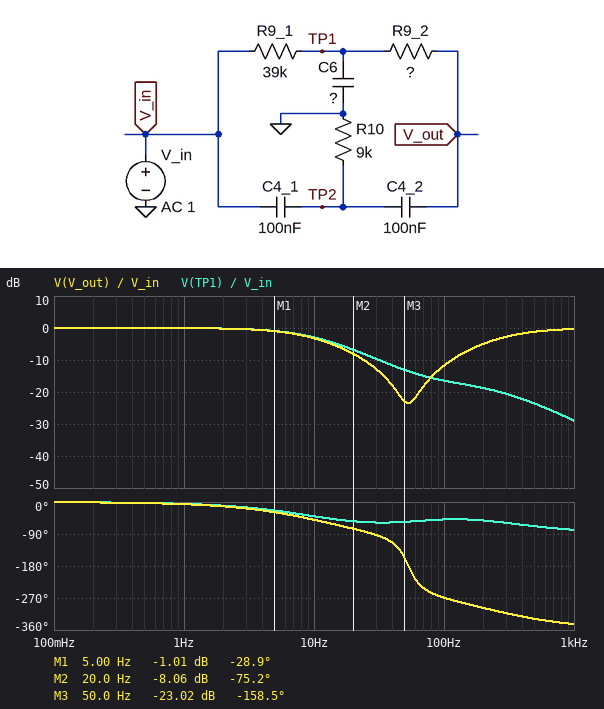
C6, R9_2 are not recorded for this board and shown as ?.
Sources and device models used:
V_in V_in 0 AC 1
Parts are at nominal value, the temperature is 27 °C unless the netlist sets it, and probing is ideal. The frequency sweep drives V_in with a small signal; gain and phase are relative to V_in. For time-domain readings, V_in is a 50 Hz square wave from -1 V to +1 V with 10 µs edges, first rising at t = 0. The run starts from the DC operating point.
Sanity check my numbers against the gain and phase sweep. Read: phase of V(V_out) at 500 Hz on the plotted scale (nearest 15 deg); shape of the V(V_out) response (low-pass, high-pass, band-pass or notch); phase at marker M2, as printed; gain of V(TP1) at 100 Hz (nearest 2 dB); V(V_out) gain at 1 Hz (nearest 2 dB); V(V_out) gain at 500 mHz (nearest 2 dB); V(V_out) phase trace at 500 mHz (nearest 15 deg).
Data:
-330 deg
notch
-75.2 deg
-16 dB
0 dB
0 dB
0 deg
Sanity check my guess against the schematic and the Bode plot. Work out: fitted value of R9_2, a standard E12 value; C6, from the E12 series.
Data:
27 kΩ
270 nF
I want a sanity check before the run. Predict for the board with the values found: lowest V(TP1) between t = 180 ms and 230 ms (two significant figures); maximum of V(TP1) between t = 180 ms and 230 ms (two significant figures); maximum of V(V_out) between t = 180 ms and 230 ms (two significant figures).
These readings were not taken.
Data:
-360 mV
360 mV
1.8 V
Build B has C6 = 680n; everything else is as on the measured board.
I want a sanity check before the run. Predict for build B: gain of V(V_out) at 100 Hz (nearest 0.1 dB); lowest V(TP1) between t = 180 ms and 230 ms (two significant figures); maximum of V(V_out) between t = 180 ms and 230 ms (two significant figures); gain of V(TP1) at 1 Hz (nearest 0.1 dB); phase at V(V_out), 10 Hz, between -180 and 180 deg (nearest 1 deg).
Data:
-10.3 dB
-180 mV
1.9 V
-0.2 dB
-71 deg
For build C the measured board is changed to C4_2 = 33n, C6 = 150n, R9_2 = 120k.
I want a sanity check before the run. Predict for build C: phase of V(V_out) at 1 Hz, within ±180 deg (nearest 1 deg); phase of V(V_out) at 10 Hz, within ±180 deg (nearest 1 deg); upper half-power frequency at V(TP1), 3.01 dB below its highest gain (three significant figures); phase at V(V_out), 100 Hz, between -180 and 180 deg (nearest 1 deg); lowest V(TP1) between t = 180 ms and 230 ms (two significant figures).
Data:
-4 deg
-38 deg
20.8 Hz
90 deg
-620 mV
